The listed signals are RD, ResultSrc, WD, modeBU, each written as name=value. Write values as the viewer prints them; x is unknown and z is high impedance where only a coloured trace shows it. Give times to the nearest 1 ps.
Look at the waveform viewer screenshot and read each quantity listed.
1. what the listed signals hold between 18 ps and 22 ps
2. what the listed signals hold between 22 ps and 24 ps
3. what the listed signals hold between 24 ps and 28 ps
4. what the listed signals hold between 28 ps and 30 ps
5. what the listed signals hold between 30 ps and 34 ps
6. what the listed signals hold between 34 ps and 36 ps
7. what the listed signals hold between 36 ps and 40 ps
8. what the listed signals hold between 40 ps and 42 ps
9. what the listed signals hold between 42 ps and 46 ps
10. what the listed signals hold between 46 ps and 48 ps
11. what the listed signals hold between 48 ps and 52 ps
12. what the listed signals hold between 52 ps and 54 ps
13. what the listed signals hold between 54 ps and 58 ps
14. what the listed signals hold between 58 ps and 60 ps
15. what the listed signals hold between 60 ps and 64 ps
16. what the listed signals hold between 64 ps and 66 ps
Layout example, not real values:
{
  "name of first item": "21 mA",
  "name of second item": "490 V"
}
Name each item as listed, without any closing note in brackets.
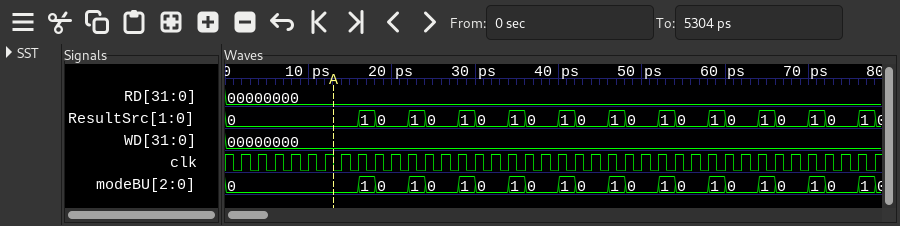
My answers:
{
  "what the listed signals hold between 18 ps and 22 ps": "RD=00000000, ResultSrc=0, WD=00000000, modeBU=0",
  "what the listed signals hold between 22 ps and 24 ps": "RD=00000000, ResultSrc=1, WD=00000000, modeBU=1",
  "what the listed signals hold between 24 ps and 28 ps": "RD=00000000, ResultSrc=0, WD=00000000, modeBU=0",
  "what the listed signals hold between 28 ps and 30 ps": "RD=00000000, ResultSrc=1, WD=00000000, modeBU=1",
  "what the listed signals hold between 30 ps and 34 ps": "RD=00000000, ResultSrc=0, WD=00000000, modeBU=0",
  "what the listed signals hold between 34 ps and 36 ps": "RD=00000000, ResultSrc=1, WD=00000000, modeBU=1",
  "what the listed signals hold between 36 ps and 40 ps": "RD=00000000, ResultSrc=0, WD=00000000, modeBU=0",
  "what the listed signals hold between 40 ps and 42 ps": "RD=00000000, ResultSrc=1, WD=00000000, modeBU=1",
  "what the listed signals hold between 42 ps and 46 ps": "RD=00000000, ResultSrc=0, WD=00000000, modeBU=0",
  "what the listed signals hold between 46 ps and 48 ps": "RD=00000000, ResultSrc=1, WD=00000000, modeBU=1",
  "what the listed signals hold between 48 ps and 52 ps": "RD=00000000, ResultSrc=0, WD=00000000, modeBU=0",
  "what the listed signals hold between 52 ps and 54 ps": "RD=00000000, ResultSrc=1, WD=00000000, modeBU=1",
  "what the listed signals hold between 54 ps and 58 ps": "RD=00000000, ResultSrc=0, WD=00000000, modeBU=0",
  "what the listed signals hold between 58 ps and 60 ps": "RD=00000000, ResultSrc=1, WD=00000000, modeBU=1",
  "what the listed signals hold between 60 ps and 64 ps": "RD=00000000, ResultSrc=0, WD=00000000, modeBU=0",
  "what the listed signals hold between 64 ps and 66 ps": "RD=00000000, ResultSrc=1, WD=00000000, modeBU=1"
}
